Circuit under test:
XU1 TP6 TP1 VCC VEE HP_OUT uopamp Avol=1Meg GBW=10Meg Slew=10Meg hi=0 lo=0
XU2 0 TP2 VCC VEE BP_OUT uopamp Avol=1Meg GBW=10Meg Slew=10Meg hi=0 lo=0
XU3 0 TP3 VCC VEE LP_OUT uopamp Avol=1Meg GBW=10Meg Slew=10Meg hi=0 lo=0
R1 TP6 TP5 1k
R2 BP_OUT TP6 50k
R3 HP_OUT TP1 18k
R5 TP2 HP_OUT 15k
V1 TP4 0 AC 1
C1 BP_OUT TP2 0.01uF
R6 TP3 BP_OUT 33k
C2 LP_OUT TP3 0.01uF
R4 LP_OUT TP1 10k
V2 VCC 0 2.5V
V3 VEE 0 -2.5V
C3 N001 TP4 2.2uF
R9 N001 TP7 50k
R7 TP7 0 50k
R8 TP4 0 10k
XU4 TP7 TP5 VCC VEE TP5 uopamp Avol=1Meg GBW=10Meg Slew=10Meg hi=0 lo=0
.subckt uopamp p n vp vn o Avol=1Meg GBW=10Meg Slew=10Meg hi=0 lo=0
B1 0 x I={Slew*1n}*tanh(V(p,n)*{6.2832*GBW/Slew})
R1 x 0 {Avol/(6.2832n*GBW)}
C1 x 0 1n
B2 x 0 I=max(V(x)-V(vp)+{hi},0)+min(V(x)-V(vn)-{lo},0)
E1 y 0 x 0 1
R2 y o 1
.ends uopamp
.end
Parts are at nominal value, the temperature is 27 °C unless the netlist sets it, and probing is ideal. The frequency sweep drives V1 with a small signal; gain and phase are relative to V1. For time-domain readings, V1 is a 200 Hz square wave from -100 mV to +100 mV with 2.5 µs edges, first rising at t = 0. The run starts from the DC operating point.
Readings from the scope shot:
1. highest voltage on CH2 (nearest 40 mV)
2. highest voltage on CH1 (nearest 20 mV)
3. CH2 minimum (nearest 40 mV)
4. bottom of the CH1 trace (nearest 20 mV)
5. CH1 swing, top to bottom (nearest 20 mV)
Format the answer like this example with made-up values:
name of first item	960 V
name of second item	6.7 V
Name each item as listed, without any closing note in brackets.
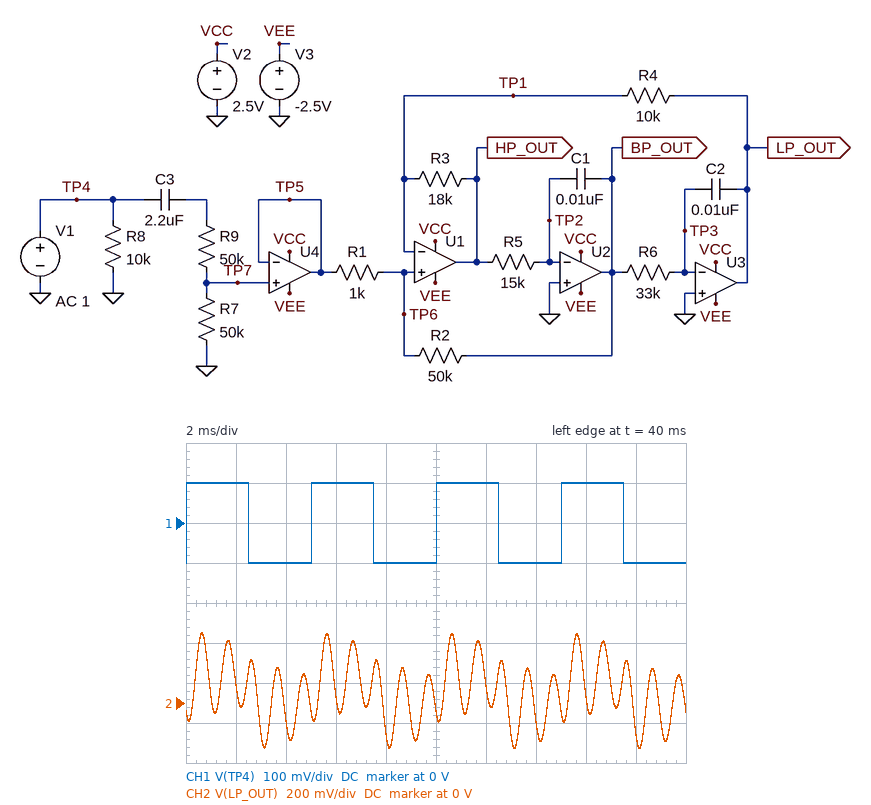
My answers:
highest voltage on CH2	360 mV
highest voltage on CH1	100 mV
CH2 minimum	-240 mV
bottom of the CH1 trace	-100 mV
CH1 swing, top to bottom	200 mV
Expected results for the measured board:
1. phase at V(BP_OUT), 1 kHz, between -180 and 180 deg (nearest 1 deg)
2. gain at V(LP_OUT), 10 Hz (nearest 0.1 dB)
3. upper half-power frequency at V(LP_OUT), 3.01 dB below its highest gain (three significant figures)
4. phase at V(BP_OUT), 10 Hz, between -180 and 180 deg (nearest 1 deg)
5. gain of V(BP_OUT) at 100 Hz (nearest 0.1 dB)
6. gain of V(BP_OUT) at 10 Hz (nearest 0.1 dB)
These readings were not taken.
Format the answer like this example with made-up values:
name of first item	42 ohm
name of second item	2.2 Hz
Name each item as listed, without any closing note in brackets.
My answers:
phase at V(BP_OUT), 1 kHz, between -180 and 180 deg	126 deg
gain at V(LP_OUT), 10 Hz	-2.4 dB
upper half-power frequency at V(LP_OUT), 3.01 dB below its highest gain	987 Hz
phase at V(BP_OUT), 10 Hz, between -180 and 180 deg	-86 deg
gain of V(BP_OUT) at 100 Hz	-15.9 dB
gain of V(BP_OUT) at 10 Hz	-36.0 dB
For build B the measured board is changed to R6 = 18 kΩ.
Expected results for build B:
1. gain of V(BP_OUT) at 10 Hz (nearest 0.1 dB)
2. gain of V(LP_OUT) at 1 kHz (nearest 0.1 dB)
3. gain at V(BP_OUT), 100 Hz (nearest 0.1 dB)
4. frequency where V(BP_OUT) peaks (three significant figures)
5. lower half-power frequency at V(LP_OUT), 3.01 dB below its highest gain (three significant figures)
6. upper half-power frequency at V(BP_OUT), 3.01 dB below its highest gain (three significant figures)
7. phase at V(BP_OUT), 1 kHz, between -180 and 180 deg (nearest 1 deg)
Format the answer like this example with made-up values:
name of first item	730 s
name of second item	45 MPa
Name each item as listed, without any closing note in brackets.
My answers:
gain of V(BP_OUT) at 10 Hz	-41.3 dB
gain of V(LP_OUT) at 1 kHz	5.4 dB
gain at V(BP_OUT), 100 Hz	-21.2 dB
frequency where V(BP_OUT) peaks	1.30 kHz
lower half-power frequency at V(LP_OUT), 3.01 dB below its highest gain	1.27 kHz
upper half-power frequency at V(BP_OUT), 3.01 dB below its highest gain	1.33 kHz
phase at V(BP_OUT), 1 kHz, between -180 and 180 deg	-95 deg
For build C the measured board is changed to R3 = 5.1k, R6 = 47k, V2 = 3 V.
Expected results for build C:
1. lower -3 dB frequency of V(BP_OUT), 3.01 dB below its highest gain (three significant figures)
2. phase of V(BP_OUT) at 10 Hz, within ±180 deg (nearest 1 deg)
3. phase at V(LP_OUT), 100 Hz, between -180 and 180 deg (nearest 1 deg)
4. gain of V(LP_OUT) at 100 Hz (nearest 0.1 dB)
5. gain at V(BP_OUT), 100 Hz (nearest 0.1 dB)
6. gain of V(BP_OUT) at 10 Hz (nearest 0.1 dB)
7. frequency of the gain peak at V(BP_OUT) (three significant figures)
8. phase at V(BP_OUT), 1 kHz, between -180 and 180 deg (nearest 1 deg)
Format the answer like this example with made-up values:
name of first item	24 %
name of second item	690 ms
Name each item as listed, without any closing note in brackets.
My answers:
lower -3 dB frequency of V(BP_OUT), 3.01 dB below its highest gain	413 Hz
phase of V(BP_OUT) at 10 Hz, within ±180 deg	-86 deg
phase at V(LP_OUT), 100 Hz, between -180 and 180 deg	-1 deg
gain of V(LP_OUT) at 100 Hz	3.7 dB
gain at V(BP_OUT), 100 Hz	-6.9 dB
gain of V(BP_OUT) at 10 Hz	-27.4 dB
frequency of the gain peak at V(BP_OUT)	428 Hz
phase at V(BP_OUT), 1 kHz, between -180 and 180 deg	92 deg
